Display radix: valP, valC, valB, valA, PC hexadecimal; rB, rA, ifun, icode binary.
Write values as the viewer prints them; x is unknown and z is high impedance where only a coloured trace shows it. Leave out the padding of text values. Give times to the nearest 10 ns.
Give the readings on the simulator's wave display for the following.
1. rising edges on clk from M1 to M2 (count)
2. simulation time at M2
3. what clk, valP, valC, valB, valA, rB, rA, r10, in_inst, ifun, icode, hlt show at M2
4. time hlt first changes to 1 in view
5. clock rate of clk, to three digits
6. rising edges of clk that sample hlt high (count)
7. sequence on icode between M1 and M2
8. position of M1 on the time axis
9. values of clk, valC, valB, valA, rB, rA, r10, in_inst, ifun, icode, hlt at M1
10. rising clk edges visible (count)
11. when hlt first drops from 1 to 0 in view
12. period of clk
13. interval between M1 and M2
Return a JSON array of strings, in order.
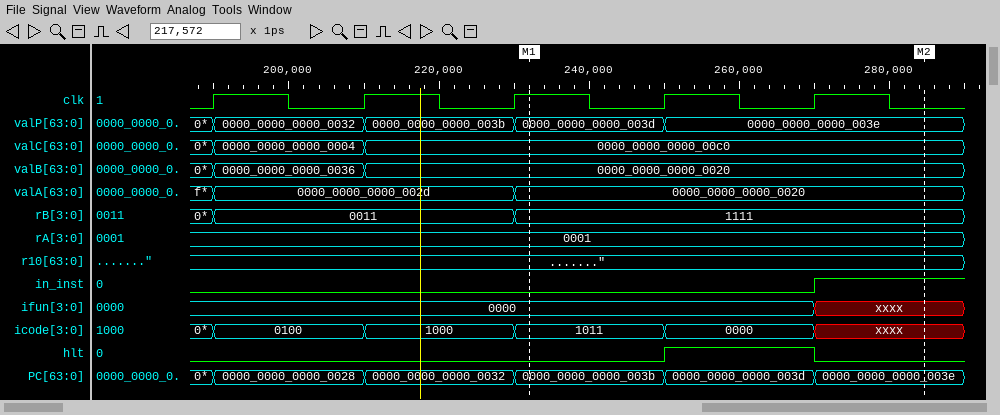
["2", "280 ns", "clk=0, valP=0000_0000_0000_003e, valC=0000_0000_0000_00c0, valB=0000_0000_0000_0020, valA=0000_0000_0000_0020, rB=1111, rA=0001, r10=\", in_inst=1, ifun=xxxx, icode=xxxx, hlt=0", "250 ns", "50.0 MHz", "1", "1011, 0000, xxxx", "230 ns", "clk=1, valC=0000_0000_0000_00c0, valB=0000_0000_0000_0020, valA=0000_0000_0000_0020, rB=1111, rA=0001, r10=\", in_inst=0, ifun=0000, icode=1011, hlt=0", "5", "270 ns", "20 ns", "50 ns"]
